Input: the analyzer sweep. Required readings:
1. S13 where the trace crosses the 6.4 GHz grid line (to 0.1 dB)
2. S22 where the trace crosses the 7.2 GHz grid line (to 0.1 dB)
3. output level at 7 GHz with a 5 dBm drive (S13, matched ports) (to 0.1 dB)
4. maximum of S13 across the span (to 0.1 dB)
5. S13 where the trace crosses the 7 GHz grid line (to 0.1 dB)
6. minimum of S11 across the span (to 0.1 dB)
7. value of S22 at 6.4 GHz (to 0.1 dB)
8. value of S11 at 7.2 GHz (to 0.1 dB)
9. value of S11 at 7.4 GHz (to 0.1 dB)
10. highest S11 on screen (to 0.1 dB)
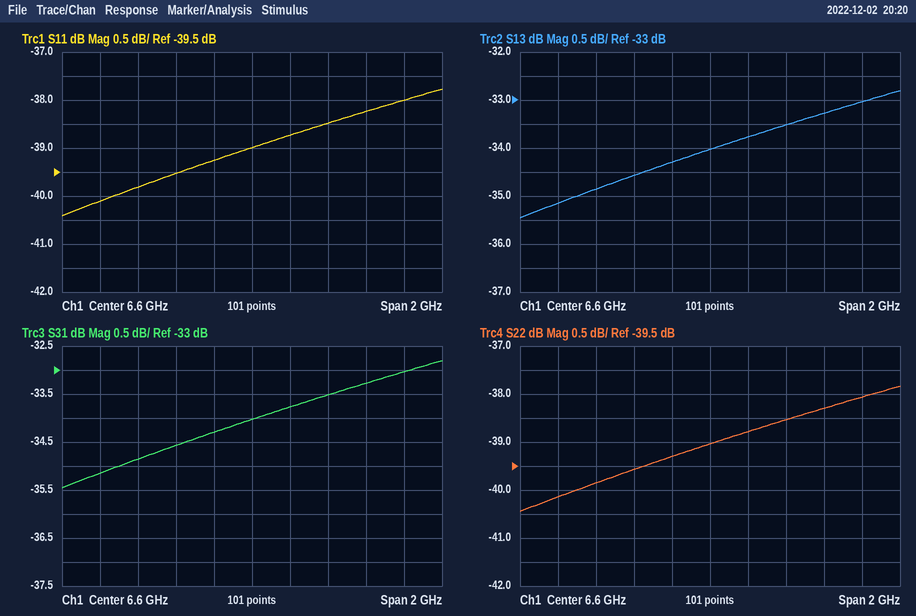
-34.3 dB
-38.3 dB
-28.5 dBm
-32.8 dB
-33.5 dB
-40.4 dB
-39.3 dB
-38.2 dB
-38.0 dB
-37.8 dB
